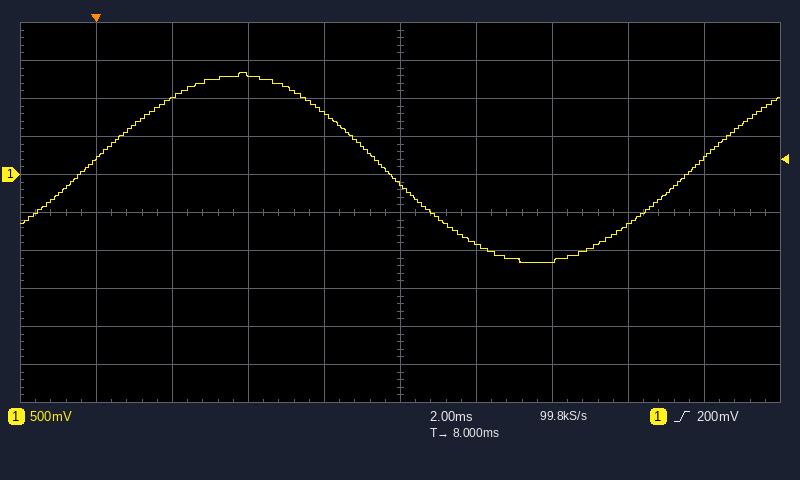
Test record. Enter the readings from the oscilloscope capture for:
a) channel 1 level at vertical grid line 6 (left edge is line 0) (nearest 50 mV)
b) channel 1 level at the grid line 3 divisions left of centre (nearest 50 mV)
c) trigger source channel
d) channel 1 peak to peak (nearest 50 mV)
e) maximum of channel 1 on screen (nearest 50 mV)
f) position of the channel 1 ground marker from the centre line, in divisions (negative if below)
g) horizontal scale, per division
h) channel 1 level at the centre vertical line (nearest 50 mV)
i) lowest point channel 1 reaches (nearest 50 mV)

-900 mV
1.00 V
channel 1
2.50 V
1.35 V
+1.0 div
2 ms
-150 mV
-1.15 V
